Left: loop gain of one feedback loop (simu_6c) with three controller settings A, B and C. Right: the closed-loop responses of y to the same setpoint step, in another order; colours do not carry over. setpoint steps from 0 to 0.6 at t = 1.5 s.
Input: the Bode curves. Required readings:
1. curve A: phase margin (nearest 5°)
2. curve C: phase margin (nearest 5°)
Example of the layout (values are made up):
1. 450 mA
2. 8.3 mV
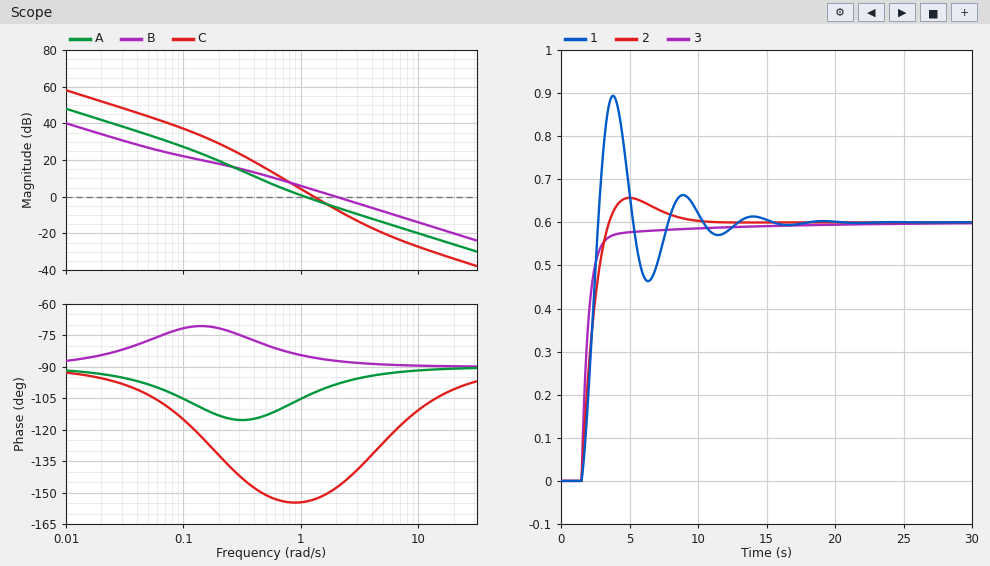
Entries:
1. 75°
2. 25°
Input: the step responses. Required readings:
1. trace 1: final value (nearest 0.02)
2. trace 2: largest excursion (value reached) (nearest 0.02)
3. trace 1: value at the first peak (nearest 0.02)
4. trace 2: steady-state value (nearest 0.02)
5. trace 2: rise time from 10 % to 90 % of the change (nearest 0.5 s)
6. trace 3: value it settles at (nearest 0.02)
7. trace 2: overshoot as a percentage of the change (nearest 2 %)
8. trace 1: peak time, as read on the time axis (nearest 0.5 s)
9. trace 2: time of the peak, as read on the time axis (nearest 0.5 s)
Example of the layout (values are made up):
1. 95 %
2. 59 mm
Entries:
1. 0.60
2. 0.66
3. 0.90
4. 0.60
5. 1.5 s
6. 0.60
7. 10 %
8. 4.0 s
9. 5.0 s
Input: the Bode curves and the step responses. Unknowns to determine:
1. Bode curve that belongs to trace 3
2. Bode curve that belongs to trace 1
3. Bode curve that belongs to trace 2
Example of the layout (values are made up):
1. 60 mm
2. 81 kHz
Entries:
1. B
2. C
3. A
